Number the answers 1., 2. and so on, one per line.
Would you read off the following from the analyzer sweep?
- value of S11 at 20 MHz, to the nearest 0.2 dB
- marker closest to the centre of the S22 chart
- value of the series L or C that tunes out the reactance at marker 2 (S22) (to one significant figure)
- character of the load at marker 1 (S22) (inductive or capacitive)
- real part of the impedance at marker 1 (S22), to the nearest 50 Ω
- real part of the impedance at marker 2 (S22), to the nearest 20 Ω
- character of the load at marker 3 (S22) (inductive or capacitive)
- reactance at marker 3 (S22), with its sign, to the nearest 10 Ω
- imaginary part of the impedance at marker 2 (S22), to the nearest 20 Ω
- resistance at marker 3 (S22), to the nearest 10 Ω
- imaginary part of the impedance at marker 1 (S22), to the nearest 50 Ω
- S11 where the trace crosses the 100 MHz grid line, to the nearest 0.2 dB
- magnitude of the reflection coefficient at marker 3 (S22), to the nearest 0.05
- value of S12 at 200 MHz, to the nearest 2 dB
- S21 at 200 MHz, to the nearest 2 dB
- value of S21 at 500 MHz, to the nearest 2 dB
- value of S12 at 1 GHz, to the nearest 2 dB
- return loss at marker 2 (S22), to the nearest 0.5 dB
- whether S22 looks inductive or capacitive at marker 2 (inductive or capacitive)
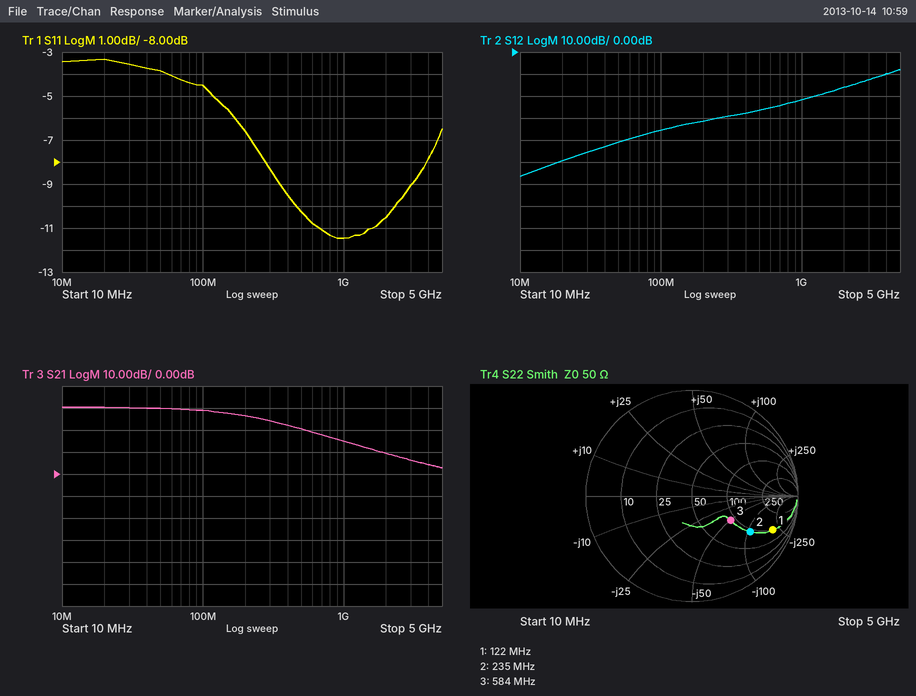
1. -3.4 dB
2. marker 3
3. 70 nH
4. capacitive
5. 100 Ω
6. 100 Ω
7. capacitive
8. -50 Ω
9. -100 Ω
10. 90 Ω
11. -200 Ω
12. -4.6 dB
13. 0.45
14. -32 dB
15. 26 dB
16. 20 dB
17. -22 dB
18. 4.0 dB
19. capacitive
